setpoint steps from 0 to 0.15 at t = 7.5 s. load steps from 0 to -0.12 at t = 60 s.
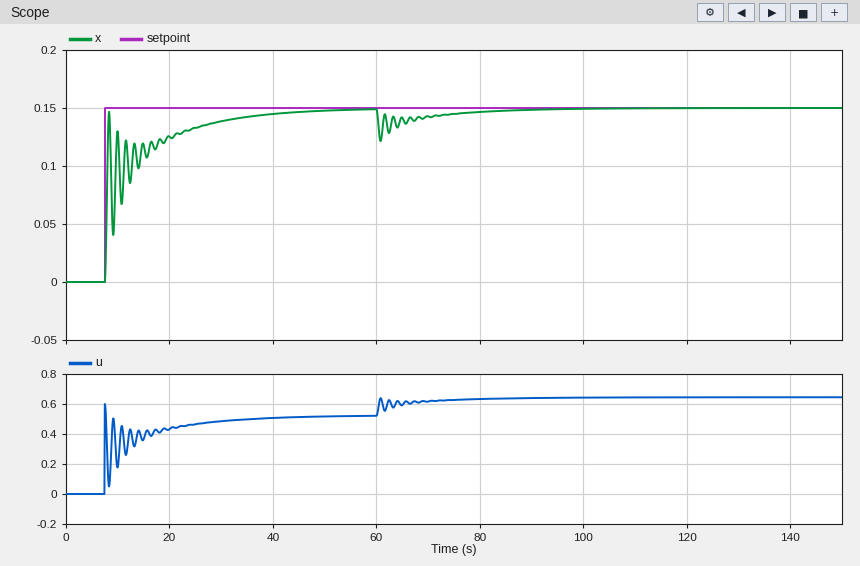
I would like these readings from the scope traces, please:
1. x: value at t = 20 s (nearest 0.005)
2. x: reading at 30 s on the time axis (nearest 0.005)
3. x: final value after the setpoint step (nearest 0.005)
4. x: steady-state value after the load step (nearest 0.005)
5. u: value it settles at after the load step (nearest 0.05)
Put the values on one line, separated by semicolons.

0.125; 0.140; 0.150; 0.150; 0.65
